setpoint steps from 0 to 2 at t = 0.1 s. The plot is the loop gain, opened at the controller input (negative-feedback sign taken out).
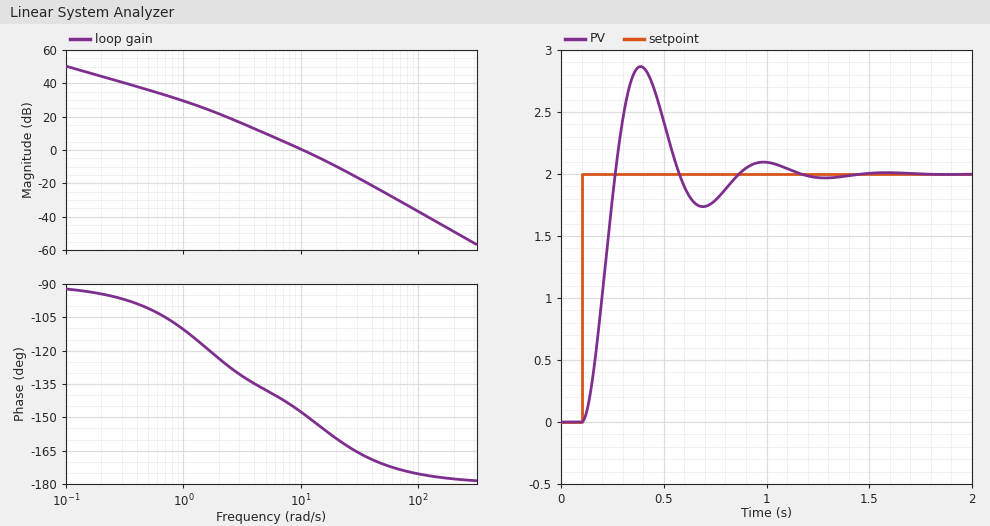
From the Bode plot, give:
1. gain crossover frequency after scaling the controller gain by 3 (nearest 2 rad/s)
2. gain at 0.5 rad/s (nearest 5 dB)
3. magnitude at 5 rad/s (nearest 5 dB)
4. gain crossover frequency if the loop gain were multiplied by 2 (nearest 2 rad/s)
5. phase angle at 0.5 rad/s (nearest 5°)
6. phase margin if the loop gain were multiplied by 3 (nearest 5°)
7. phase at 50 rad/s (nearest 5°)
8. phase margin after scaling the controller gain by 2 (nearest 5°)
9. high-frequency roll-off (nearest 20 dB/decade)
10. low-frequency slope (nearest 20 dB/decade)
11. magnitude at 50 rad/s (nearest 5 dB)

20 rad/s
35 dB
10 dB
16 rad/s
-100°
20°
-170°
25°
-40 dB/decade
-20 dB/decade
-25 dB
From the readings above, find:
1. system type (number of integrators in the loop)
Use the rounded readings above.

1
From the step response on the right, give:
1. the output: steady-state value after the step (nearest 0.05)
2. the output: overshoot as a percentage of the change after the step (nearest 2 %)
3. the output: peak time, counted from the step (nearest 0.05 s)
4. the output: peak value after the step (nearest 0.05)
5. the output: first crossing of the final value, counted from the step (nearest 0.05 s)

2.00
44 %
0.30 s
2.85
0.15 s
